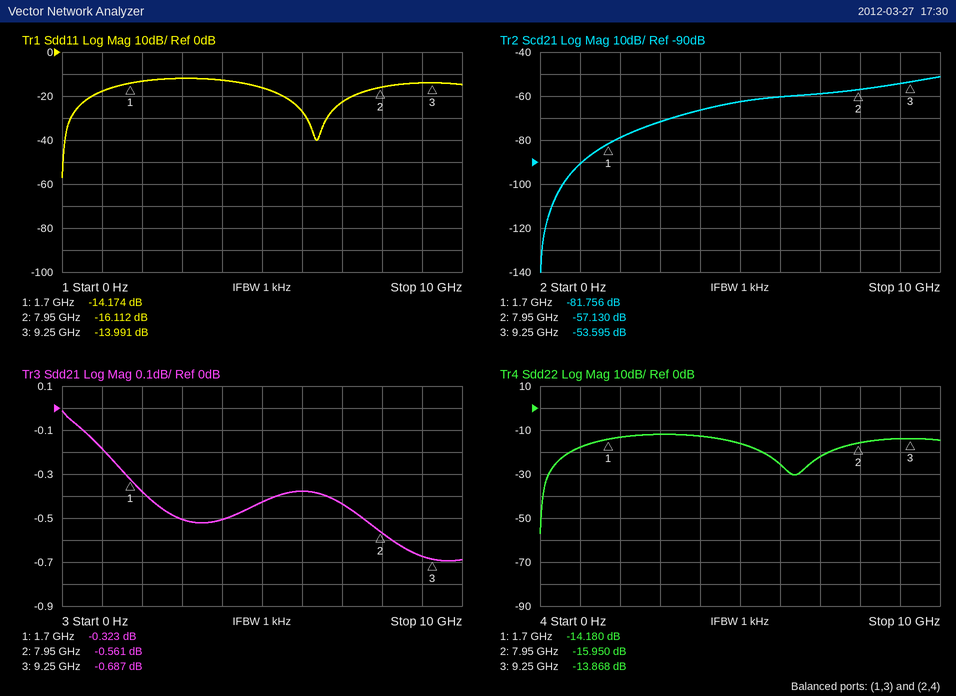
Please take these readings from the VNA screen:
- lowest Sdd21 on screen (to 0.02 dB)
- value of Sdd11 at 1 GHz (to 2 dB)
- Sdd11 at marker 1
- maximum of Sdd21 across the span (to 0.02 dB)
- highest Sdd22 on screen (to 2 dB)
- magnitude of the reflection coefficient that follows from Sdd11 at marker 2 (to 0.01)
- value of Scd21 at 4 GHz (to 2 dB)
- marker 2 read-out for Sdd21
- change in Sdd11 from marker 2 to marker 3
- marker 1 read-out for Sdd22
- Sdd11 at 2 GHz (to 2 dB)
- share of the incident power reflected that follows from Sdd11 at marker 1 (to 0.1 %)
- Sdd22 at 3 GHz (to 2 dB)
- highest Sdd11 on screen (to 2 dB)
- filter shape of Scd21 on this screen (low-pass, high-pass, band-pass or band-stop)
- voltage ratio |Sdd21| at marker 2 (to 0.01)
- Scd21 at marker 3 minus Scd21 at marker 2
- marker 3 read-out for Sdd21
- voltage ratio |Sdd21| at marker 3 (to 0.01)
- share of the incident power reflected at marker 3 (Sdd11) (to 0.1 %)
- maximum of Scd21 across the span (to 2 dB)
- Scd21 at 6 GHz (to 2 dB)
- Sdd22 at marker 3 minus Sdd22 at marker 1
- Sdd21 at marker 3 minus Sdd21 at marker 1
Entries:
-0.70 dB
-18 dB
-14.174 dB
-0.02 dB
-12 dB
0.16
-66 dB
-0.561 dB
2.121 dB
-14.180 dB
-14 dB
3.8 %
-12 dB
-12 dB
high-pass
0.94
3.535 dB
-0.687 dB
0.92
4.0 %
-52 dB
-60 dB
0.312 dB
-0.364 dB
